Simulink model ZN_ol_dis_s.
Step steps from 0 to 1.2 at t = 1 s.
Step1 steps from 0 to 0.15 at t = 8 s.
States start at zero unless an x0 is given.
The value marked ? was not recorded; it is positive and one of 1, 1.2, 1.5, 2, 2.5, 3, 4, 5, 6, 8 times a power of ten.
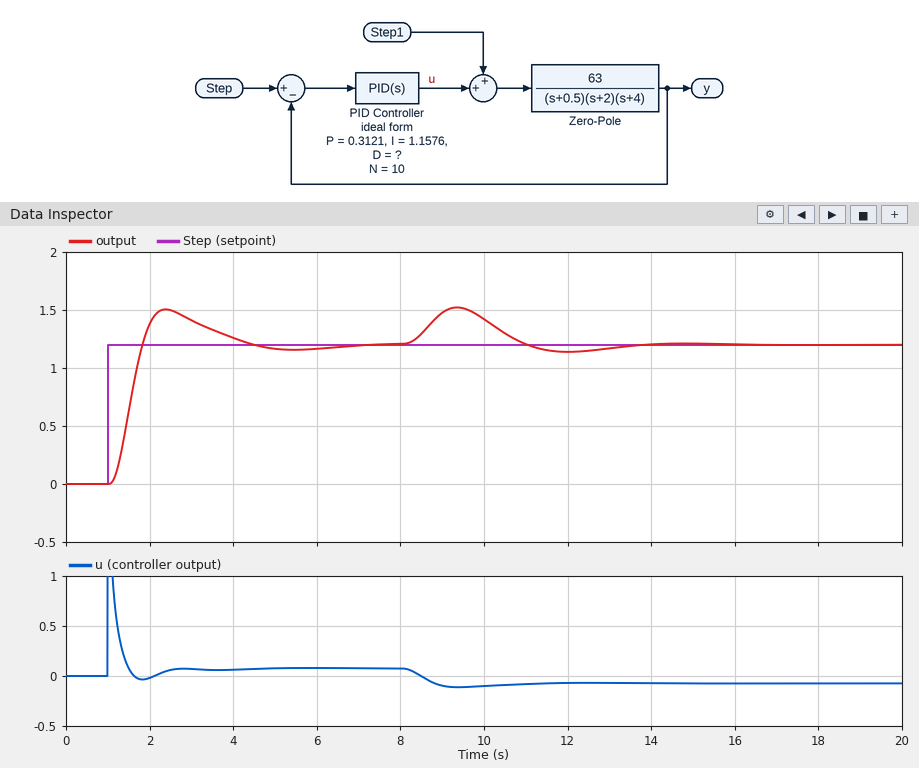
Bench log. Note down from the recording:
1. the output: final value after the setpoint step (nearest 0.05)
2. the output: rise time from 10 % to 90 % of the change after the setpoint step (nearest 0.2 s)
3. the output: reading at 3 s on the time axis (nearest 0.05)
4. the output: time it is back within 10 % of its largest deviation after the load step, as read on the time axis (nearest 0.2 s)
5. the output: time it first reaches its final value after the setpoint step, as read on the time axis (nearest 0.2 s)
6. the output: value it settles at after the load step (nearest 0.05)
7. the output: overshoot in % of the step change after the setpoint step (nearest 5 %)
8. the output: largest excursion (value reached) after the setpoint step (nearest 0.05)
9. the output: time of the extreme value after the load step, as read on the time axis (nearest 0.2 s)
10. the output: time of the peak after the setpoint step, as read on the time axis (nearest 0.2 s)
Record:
1.20
0.6 s
1.40
13.0 s
1.8 s
1.20
25 %
1.50
9.4 s
2.4 s
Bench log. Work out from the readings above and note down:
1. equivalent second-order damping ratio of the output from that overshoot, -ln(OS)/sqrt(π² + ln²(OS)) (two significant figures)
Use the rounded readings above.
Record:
0.40
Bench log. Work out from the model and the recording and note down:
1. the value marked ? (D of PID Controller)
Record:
0.5
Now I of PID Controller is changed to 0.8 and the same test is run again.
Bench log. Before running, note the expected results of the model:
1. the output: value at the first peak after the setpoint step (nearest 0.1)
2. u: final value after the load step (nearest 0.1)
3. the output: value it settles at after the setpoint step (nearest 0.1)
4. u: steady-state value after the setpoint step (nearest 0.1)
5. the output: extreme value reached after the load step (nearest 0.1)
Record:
1.4
-0.1
1.2
0.1
1.5
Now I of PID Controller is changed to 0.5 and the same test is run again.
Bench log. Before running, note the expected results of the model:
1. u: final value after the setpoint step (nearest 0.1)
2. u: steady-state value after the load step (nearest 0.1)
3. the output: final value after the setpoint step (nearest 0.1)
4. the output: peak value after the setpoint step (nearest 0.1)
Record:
0.1
-0.1
1.2
1.3
